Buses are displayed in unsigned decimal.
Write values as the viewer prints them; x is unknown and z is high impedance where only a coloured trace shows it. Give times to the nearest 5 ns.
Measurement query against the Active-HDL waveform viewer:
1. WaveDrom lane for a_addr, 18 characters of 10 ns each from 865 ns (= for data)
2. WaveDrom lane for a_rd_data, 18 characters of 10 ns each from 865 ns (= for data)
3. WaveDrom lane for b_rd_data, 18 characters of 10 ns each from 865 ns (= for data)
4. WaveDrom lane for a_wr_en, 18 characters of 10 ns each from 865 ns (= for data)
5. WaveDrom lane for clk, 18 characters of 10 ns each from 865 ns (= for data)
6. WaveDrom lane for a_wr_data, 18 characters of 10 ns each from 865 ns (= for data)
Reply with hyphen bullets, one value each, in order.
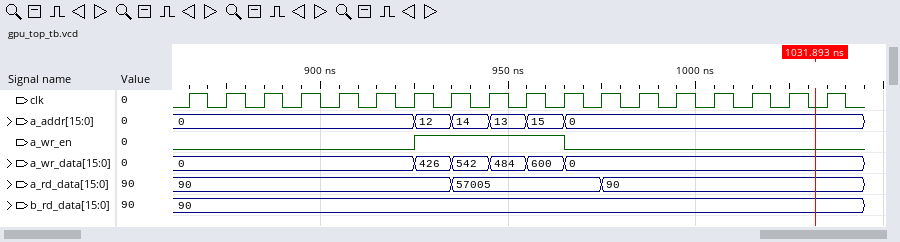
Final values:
- {name: 'a_addr', wave: '=.....=====.......', data: '0 12 14 13 15 0'}
- {name: 'a_rd_data', wave: '=......=...=......', data: '90 57005 90'}
- {name: 'b_rd_data', wave: '=.................', data: '90'}
- {name: 'a_wr_en', wave: '0.....1...0.......'}
- {name: 'clk', wave: 'p.................'}
- {name: 'a_wr_data', wave: '=.....=====.......', data: '0 426 542 484 600 0'}
